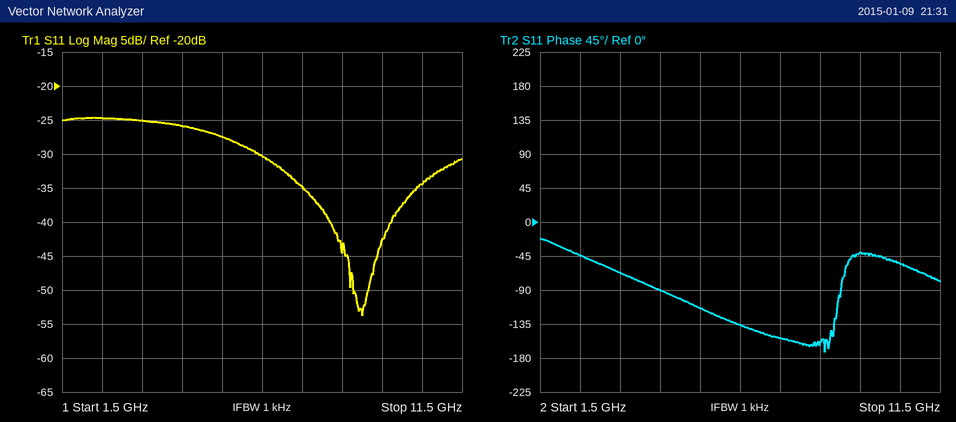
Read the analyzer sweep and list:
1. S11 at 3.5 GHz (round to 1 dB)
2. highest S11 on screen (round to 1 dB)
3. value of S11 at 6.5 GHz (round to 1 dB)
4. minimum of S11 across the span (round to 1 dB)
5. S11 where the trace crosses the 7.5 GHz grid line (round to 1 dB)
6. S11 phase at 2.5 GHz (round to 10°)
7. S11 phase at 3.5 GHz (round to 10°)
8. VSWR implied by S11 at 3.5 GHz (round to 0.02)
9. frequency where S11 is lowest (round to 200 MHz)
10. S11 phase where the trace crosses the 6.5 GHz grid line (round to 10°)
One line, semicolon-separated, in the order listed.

-25 dB; -25 dB; -30 dB; -54 dB; -35 dB; -40°; -70°; 1.12; 9.0 GHz; -140°
